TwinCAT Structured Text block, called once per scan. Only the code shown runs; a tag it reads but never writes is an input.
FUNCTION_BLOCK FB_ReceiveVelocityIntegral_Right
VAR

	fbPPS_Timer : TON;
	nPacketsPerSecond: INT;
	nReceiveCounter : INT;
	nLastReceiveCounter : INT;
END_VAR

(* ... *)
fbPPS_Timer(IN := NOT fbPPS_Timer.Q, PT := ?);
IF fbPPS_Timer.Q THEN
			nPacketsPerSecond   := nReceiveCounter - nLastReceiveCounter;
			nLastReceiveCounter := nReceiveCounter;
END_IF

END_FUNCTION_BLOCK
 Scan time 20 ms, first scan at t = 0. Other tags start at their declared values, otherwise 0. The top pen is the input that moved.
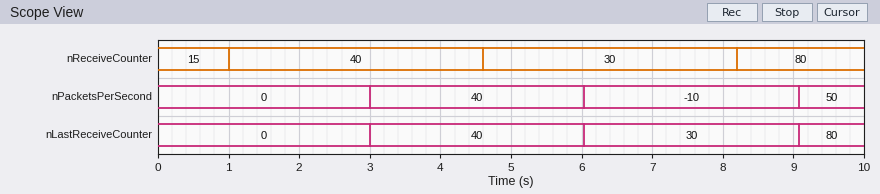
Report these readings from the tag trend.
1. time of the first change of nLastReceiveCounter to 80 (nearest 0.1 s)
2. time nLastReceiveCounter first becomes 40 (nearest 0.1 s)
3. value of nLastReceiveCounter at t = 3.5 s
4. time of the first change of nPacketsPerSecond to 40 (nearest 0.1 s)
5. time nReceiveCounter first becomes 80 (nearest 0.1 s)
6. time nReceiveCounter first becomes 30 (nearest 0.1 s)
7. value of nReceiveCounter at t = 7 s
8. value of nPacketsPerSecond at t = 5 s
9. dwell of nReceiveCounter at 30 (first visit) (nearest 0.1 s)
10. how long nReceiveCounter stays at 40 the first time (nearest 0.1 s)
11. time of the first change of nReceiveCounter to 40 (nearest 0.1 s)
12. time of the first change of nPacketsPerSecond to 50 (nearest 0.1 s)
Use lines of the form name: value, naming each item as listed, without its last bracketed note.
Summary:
time of the first change of nLastReceiveCounter to 80: 9.1 s
time nLastReceiveCounter first becomes 40: 3.0 s
value of nLastReceiveCounter at t = 3.5 s: 40
time of the first change of nPacketsPerSecond to 40: 3.0 s
time nReceiveCounter first becomes 80: 8.2 s
time nReceiveCounter first becomes 30: 4.6 s
value of nReceiveCounter at t = 7 s: 30
value of nPacketsPerSecond at t = 5 s: 40
dwell of nReceiveCounter at 30 (first visit): 3.6 s
how long nReceiveCounter stays at 40 the first time: 3.6 s
time of the first change of nReceiveCounter to 40: 1.0 s
time of the first change of nPacketsPerSecond to 50: 9.1 s
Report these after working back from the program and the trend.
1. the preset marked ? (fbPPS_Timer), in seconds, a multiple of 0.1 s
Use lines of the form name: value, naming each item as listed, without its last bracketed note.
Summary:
the preset marked ? (fbPPS_Timer), in seconds, a multiple of 0.1 s: 3.0 s
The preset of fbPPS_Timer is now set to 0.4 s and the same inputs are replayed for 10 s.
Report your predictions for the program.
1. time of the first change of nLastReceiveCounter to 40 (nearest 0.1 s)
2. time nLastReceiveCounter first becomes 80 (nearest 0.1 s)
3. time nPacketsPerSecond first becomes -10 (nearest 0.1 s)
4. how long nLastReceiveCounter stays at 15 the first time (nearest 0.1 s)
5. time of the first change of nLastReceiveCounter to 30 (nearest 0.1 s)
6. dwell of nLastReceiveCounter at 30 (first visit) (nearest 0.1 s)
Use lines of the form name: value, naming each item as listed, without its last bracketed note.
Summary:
time of the first change of nLastReceiveCounter to 40: 1.3 s
time nLastReceiveCounter first becomes 80: 8.3 s
time nPacketsPerSecond first becomes -10: 4.8 s
how long nLastReceiveCounter stays at 15 the first time: 0.9 s
time of the first change of nLastReceiveCounter to 30: 4.8 s
dwell of nLastReceiveCounter at 30 (first visit): 3.5 s
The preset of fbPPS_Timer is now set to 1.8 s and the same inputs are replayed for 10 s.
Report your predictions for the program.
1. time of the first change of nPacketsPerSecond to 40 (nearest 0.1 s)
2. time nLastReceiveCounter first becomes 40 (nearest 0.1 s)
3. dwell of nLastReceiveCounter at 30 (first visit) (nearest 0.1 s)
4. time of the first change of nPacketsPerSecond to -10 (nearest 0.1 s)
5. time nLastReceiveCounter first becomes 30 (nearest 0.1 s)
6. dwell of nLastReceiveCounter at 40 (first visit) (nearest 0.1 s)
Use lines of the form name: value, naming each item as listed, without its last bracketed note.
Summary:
time of the first change of nPacketsPerSecond to 40: 1.8 s
time nLastReceiveCounter first becomes 40: 1.8 s
dwell of nLastReceiveCounter at 30 (first visit): 3.7 s
time of the first change of nPacketsPerSecond to -10: 5.5 s
time nLastReceiveCounter first becomes 30: 5.5 s
dwell of nLastReceiveCounter at 40 (first visit): 3.7 s
